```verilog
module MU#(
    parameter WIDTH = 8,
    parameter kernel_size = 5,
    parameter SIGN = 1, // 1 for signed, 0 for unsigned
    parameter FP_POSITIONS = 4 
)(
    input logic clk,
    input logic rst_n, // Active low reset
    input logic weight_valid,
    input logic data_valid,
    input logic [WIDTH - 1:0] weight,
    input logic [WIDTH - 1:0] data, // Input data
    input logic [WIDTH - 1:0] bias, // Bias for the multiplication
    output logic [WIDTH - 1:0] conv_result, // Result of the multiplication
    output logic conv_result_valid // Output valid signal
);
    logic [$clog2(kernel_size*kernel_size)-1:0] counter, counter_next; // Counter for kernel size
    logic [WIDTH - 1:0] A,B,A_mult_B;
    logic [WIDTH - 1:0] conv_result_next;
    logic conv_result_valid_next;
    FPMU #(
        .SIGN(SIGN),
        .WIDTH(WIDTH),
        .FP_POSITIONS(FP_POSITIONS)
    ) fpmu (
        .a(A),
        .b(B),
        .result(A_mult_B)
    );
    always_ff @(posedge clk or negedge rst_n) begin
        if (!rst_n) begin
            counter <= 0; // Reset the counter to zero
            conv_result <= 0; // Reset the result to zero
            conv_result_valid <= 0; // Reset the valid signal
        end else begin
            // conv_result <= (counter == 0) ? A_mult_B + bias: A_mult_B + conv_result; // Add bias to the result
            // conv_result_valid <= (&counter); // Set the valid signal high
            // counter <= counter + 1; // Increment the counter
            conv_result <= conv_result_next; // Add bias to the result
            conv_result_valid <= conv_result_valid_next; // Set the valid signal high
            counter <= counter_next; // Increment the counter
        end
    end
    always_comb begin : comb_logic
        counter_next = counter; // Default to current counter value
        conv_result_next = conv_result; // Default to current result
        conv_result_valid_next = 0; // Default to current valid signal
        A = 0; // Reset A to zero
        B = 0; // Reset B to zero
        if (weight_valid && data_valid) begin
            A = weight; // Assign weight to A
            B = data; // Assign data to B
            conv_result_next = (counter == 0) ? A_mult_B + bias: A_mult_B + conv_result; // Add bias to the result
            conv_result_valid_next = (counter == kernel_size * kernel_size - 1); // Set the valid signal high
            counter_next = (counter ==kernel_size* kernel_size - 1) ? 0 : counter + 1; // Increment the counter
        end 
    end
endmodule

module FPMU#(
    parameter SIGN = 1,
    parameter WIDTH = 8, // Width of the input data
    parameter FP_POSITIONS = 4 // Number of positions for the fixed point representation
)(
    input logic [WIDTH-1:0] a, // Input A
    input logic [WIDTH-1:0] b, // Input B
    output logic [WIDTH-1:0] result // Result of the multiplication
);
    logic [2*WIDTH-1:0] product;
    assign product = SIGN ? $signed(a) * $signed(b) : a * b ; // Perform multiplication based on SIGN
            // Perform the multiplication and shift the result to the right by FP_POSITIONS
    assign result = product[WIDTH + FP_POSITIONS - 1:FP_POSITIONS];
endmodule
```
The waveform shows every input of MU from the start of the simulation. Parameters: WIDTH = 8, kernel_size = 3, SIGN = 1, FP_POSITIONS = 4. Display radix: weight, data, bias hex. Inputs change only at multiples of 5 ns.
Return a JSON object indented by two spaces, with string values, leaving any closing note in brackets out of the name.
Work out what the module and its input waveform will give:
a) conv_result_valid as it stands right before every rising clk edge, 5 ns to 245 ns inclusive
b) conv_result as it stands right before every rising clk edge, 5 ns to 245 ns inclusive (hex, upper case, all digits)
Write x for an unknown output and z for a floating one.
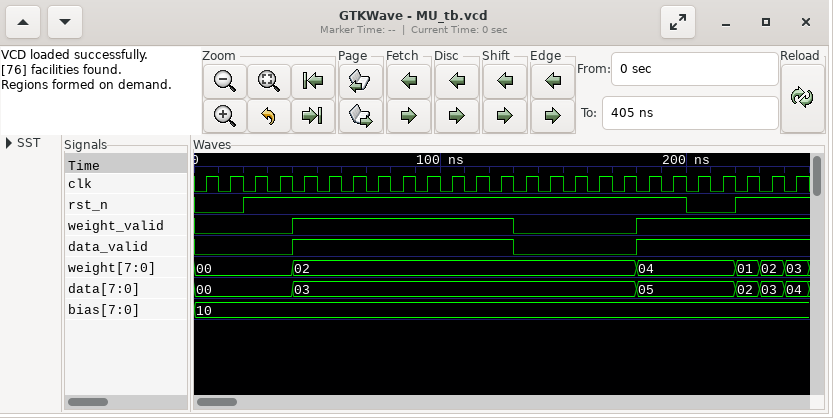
{
  "conv_result_valid as it stands right before every rising clk edge, 5 ns to 245 ns inclusive": "0 0 0 0 0 0 0 0 0 0 0 0 0 1 0 0 0 0 0 0 0 0 0 0 0",
  "conv_result as it stands right before every rising clk edge, 5 ns to 245 ns inclusive": "00, 00, 00, 00, 00, 10, 10, 10, 10, 10, 10, 10, 10, 10, 10, 10, 10, 10, 10, 11, 00, 00, 00, 10, 10"
}
